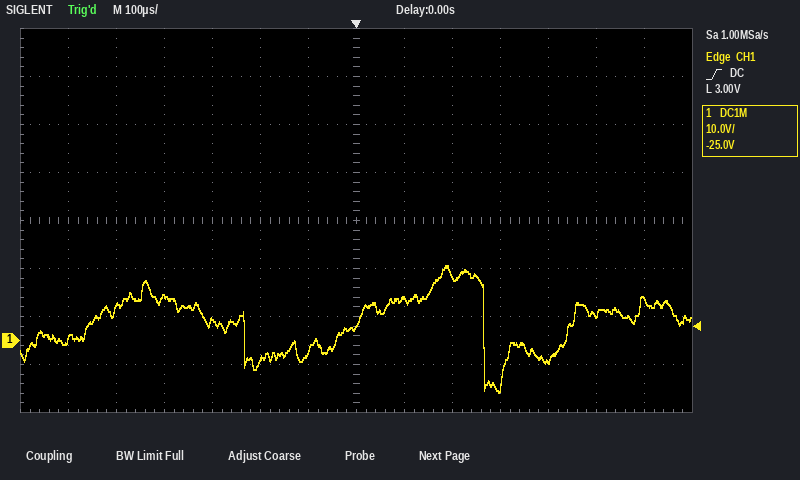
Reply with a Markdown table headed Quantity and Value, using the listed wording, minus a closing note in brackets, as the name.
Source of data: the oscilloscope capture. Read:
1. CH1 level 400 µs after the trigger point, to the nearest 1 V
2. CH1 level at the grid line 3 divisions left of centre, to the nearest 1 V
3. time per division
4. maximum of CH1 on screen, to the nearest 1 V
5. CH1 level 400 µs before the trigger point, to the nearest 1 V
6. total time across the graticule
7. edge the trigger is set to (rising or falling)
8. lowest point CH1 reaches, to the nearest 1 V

| Quantity | Value |
|---|---|
| CH1 level 400 µs after the trigger point, to the nearest 1 V | -4 V |
| CH1 level at the grid line 3 divisions left of centre, to the nearest 1 V | 4 V |
| time per division | 100 µs |
| maximum of CH1 on screen, to the nearest 1 V | 16 V |
| CH1 level 400 µs before the trigger point, to the nearest 1 V | 9 V |
| total time across the graticule | 1.4 ms |
| edge the trigger is set to | rising |
| lowest point CH1 reaches, to the nearest 1 V | -11 V |
